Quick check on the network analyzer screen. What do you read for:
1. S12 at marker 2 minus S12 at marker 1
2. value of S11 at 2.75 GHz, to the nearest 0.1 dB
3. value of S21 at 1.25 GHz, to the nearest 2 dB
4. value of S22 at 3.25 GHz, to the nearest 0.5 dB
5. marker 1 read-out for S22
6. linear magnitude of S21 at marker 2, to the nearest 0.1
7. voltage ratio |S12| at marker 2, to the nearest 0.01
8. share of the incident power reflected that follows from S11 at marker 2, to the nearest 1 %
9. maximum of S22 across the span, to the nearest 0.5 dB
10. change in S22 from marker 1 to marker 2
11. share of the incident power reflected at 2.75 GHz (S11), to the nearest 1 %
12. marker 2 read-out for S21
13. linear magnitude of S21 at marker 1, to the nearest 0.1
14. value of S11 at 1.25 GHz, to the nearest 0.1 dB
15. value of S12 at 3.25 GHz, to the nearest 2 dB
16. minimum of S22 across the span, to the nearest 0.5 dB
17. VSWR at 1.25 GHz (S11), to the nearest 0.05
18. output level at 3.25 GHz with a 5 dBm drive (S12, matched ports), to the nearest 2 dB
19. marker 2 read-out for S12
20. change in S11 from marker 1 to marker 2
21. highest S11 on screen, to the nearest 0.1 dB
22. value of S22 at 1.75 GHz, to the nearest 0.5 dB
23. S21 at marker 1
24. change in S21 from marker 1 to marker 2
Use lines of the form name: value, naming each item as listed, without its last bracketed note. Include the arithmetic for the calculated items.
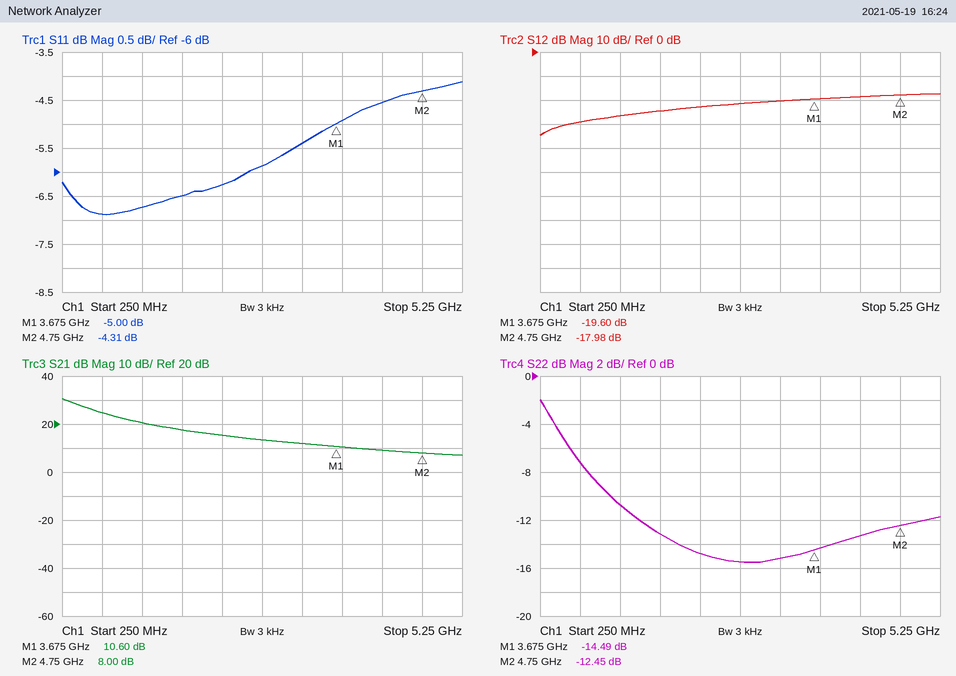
S12 at marker 2 minus S12 at marker 1: -17.98 − (-19.6) = 1.62 dB
value of S11 at 2.75 GHz, to the nearest 0.1 dB: -5.9 dB
value of S21 at 1.25 GHz, to the nearest 2 dB: 20 dB
value of S22 at 3.25 GHz, to the nearest 0.5 dB: -15.0 dB
marker 1 read-out for S22: -14.49 dB
linear magnitude of S21 at marker 2, to the nearest 0.1: 10^(8/20) ≈ 2.5
voltage ratio |S12| at marker 2, to the nearest 0.01: 10^(-17.98/20) ≈ 0.13
share of the incident power reflected that follows from S11 at marker 2, to the nearest 1 %: 10^(-4.31/10) ≈ 37 %
maximum of S22 across the span, to the nearest 0.5 dB: -2.0 dB
change in S22 from marker 1 to marker 2: -12.45 − (-14.49) = 2.04 dB
share of the incident power reflected at 2.75 GHz (S11), to the nearest 1 %: 10^(-5.9/10) ≈ 26 %
marker 2 read-out for S21: 8.00 dB
linear magnitude of S21 at marker 1, to the nearest 0.1: 10^(10.6/20) ≈ 3.4
value of S11 at 1.25 GHz, to the nearest 0.1 dB: -6.7 dB
value of S12 at 3.25 GHz, to the nearest 2 dB: -20 dB
minimum of S22 across the span, to the nearest 0.5 dB: -15.5 dB
VSWR at 1.25 GHz (S11), to the nearest 0.05: |Γ| = 10^(-6.7/20) = 0.4624; VSWR = (1 + 0.4624)/(1 − 0.4624) ≈ 2.72, so 2.70 to the nearest 0.05
output level at 3.25 GHz with a 5 dBm drive (S12, matched ports), to the nearest 2 dB: 5 dBm + (-20 dB) = -16 dBm
marker 2 read-out for S12: -17.98 dB
change in S11 from marker 1 to marker 2: -4.31 − (-5) = 0.69 dB
highest S11 on screen, to the nearest 0.1 dB: -4.1 dB
value of S22 at 1.75 GHz, to the nearest 0.5 dB: -13.0 dB
S21 at marker 1: 10.60 dB
change in S21 from marker 1 to marker 2: 8 − (10.6) = -2.60 dB
